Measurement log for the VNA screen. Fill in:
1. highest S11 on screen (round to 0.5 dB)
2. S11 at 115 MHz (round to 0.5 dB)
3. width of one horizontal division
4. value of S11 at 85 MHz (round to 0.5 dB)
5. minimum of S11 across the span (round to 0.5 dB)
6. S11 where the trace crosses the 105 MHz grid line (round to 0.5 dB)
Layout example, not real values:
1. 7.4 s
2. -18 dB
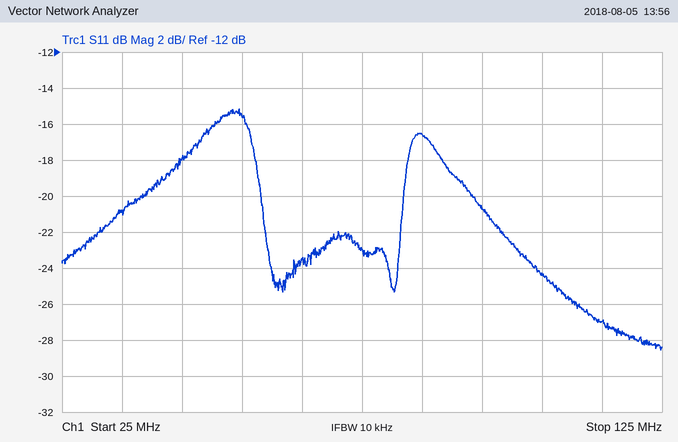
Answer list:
1. -15.0 dB
2. -27.0 dB
3. 10 MHz
4. -16.5 dB
5. -28.5 dB
6. -24.5 dB
